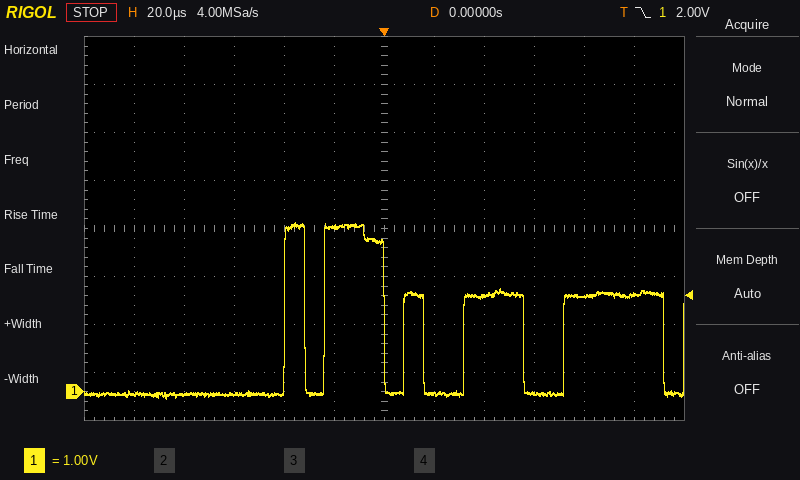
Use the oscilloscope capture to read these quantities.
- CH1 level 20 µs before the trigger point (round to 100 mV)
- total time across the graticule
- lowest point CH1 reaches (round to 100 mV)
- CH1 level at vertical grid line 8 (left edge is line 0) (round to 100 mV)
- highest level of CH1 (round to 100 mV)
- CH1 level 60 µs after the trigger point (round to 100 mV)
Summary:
3.4 V
240 µs
-100 mV
2.0 V
3.5 V
0.0 V
